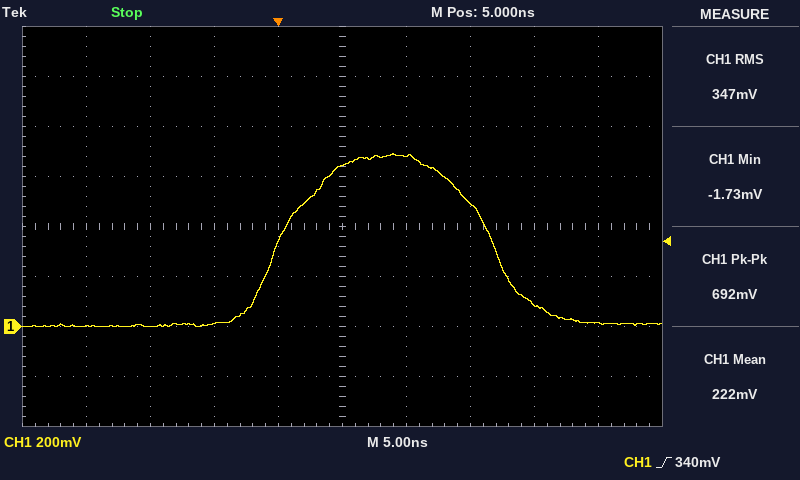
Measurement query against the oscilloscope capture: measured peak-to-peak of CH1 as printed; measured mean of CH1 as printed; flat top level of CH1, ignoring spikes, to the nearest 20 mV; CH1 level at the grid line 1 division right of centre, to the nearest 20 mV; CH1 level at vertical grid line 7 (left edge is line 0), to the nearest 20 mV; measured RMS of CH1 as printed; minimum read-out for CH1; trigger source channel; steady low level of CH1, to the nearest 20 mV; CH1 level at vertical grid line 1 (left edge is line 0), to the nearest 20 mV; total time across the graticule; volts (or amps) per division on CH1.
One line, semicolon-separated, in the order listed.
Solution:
692 mV; 222 mV; 680 mV; 680 mV; 500 mV; 347 mV; -1.73 mV; CH1; 0 mV; 0 mV; 50 ns; 200 mV
